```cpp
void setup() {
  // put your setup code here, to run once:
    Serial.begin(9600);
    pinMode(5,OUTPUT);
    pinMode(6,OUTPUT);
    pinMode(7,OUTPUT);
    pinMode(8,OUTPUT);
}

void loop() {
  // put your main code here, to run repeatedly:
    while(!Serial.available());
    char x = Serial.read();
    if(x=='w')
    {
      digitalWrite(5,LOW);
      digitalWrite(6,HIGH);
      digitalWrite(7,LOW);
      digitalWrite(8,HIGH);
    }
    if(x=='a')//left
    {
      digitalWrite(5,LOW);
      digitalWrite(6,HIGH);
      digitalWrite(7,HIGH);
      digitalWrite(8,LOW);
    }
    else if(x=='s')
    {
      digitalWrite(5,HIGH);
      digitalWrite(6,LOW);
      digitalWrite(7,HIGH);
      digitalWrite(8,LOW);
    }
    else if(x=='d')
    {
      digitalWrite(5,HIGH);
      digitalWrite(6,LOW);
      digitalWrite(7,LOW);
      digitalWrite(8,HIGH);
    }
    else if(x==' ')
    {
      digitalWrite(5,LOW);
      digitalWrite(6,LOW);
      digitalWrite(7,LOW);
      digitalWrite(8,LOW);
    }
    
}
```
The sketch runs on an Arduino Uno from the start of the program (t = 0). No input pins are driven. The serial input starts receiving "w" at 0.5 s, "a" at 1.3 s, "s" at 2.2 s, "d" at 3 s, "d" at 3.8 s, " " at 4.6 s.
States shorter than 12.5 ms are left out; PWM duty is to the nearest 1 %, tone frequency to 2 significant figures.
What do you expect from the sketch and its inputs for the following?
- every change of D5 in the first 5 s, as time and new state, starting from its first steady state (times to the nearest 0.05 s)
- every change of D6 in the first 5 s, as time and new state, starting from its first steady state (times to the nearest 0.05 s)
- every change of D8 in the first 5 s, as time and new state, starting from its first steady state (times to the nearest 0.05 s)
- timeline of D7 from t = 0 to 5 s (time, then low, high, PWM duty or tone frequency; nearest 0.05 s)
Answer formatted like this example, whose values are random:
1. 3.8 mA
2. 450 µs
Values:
1. 0 s low; 2.2 s high; 4.6 s low
2. 0 s low; 0.5 s high; 2.2 s low
3. 0 s low; 0.5 s high; 1.3 s low; 3 s high; 4.6 s low
4. 0 s low; 1.3 s high; 3 s low
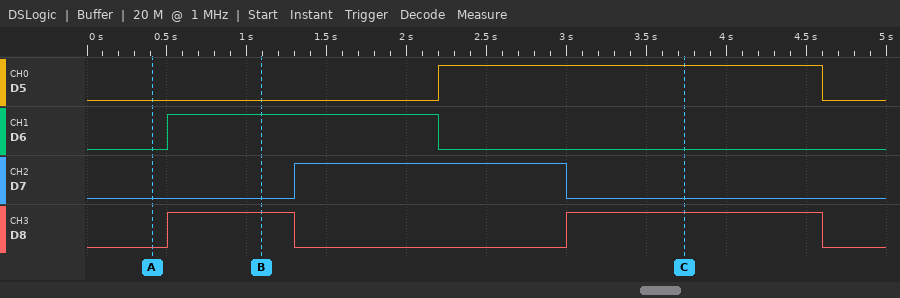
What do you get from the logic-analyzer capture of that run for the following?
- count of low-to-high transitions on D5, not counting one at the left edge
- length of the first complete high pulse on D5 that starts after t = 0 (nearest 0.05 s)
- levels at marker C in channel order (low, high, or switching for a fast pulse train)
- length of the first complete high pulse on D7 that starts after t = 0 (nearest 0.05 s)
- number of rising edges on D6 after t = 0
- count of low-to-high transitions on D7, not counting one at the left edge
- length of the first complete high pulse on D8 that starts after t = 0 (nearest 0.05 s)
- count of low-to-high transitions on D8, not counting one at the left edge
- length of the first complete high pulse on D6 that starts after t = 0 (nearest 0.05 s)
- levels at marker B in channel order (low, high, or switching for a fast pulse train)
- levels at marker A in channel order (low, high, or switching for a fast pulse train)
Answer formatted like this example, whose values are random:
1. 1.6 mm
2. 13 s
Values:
1. 1
2. 2.40 s
3. D5 high, D6 low, D7 low, D8 high
4. 1.70 s
5. 1
6. 1
7. 0.80 s
8. 2
9. 1.70 s
10. D5 low, D6 high, D7 low, D8 high
11. D5 low, D6 low, D7 low, D8 low
